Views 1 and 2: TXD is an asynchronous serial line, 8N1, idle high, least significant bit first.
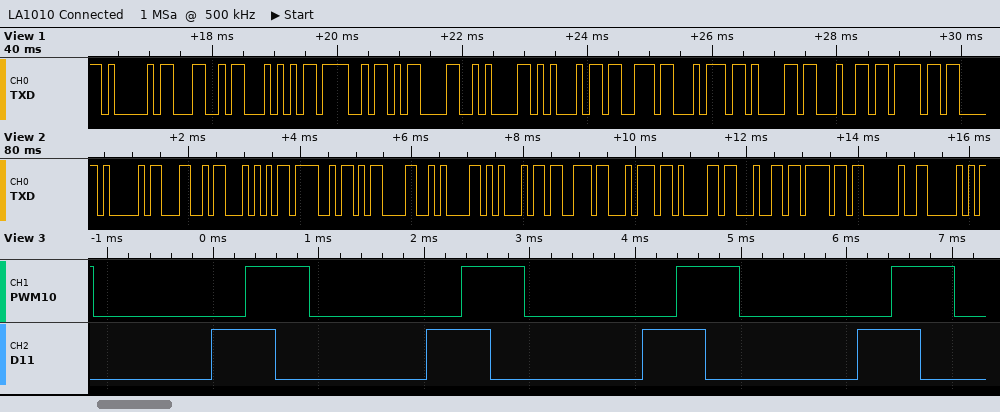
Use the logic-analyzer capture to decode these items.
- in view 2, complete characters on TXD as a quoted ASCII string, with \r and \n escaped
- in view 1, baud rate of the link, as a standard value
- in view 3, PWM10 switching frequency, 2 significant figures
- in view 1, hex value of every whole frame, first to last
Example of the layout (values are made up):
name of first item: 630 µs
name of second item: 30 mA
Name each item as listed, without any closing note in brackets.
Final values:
in view 2, complete characters on TXD as a quoted ASCII string, with \r and \n escaped: "ALTO\r\nEstado P"
in view 1, baud rate of the link, as a standard value: 9600 baud
in view 3, PWM10 switching frequency, 2 significant figures: 490 Hz
in view 1, hex value of every whole frame, first to last: 0x41 0x4C 0x54 0x4F 0x0D 0x0A 0x45 0x73 0x74 0x61 0x64 0x6F
